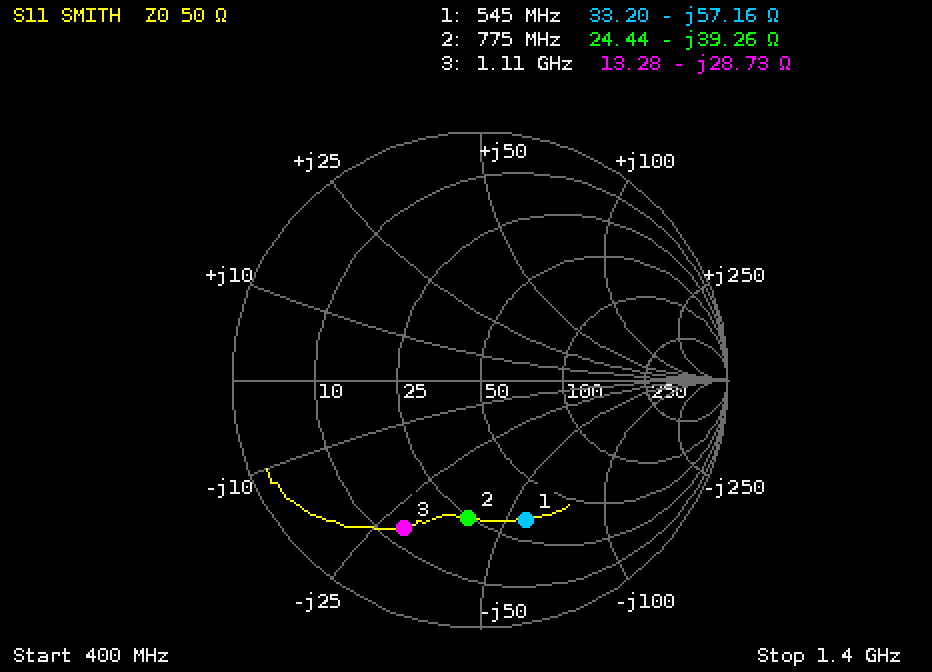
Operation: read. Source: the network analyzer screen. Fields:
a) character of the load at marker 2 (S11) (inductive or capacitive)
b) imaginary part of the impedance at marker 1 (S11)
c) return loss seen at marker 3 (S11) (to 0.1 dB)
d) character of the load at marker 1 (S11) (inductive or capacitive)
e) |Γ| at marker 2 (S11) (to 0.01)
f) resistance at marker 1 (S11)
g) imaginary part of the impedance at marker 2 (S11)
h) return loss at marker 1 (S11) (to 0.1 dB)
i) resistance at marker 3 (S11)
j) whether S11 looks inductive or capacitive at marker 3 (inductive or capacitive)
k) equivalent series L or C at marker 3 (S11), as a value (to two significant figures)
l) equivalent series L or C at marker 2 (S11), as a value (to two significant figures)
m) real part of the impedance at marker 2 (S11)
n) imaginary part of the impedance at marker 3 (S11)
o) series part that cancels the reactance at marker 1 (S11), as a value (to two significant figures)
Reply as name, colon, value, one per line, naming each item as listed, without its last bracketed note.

character of the load at marker 2 (S11): capacitive
imaginary part of the impedance at marker 1: -57.16 Ω
return loss seen at marker 3 (S11): 3.5 dB
character of the load at marker 1 (S11): capacitive
|Γ| at marker 2 (S11): 0.56
resistance at marker 1: 33.20 Ω
imaginary part of the impedance at marker 2: -39.26 Ω
return loss at marker 1 (S11): 4.6 dB
resistance at marker 3: 13.28 Ω
whether S11 looks inductive or capacitive at marker 3: capacitive
equivalent series L or C at marker 3 (S11), as a value: 5.0 pF
equivalent series L or C at marker 2 (S11), as a value: 5.2 pF
real part of the impedance at marker 2: 24.44 Ω
imaginary part of the impedance at marker 3: -28.73 Ω
series part that cancels the reactance at marker 1 (S11), as a value: 17 nH
